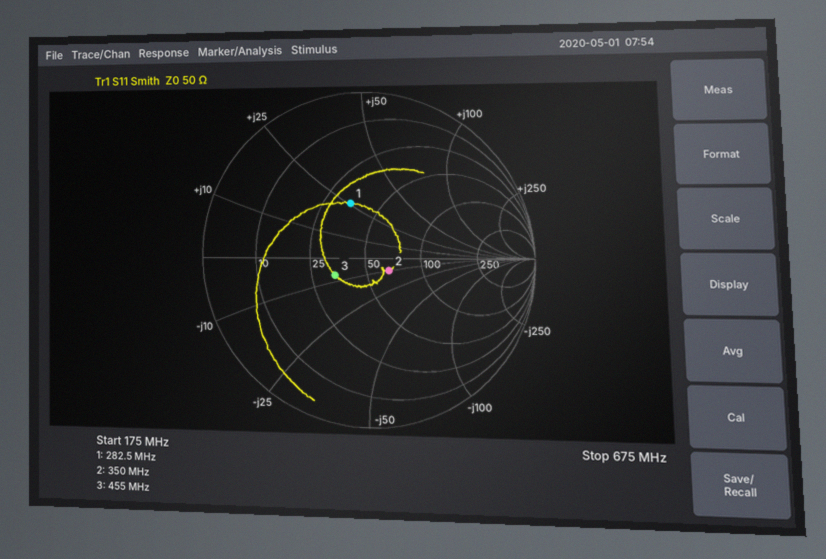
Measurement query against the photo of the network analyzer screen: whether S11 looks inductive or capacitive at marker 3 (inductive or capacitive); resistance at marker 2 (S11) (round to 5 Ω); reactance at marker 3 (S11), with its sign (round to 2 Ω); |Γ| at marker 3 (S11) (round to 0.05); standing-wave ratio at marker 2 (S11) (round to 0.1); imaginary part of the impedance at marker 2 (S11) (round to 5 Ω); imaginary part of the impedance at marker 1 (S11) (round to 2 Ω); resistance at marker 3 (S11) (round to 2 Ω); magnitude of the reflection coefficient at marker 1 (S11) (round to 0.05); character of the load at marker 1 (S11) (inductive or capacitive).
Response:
capacitive
65 Ω
-8 Ω
0.20
1.4
-10 Ω
+26 Ω
34 Ω
0.35
inductive
